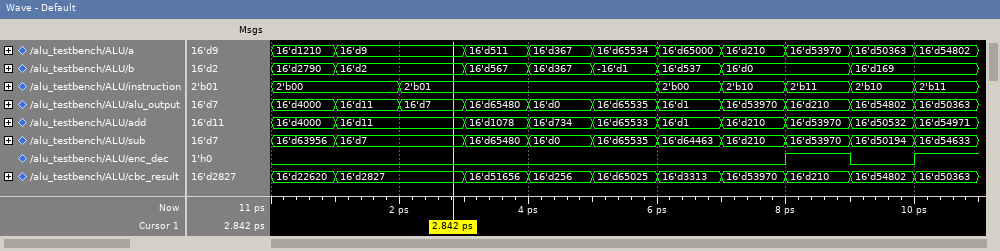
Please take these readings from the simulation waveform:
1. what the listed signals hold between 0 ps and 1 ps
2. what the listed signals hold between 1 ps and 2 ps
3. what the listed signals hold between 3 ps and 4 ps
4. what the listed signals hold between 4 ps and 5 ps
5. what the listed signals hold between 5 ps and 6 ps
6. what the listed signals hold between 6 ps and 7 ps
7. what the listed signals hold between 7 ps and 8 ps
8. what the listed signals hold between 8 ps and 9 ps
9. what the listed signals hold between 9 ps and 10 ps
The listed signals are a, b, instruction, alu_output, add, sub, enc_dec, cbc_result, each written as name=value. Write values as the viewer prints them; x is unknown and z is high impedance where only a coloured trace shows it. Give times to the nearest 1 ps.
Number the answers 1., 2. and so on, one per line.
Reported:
1. a=16'd1210, b=16'd2790, instruction=2'b00, alu_output=16'd4000, add=16'd4000, sub=16'd63956, enc_dec=0, cbc_result=16'd22620
2. a=16'd9, b=16'd2, instruction=2'b00, alu_output=16'd11, add=16'd11, sub=16'd7, enc_dec=0, cbc_result=16'd2827
3. a=16'd511, b=16'd567, instruction=2'b01, alu_output=16'd65480, add=16'd1078, sub=16'd65480, enc_dec=0, cbc_result=16'd51656
4. a=16'd367, b=16'd367, instruction=2'b01, alu_output=16'd0, add=16'd734, sub=16'd0, enc_dec=0, cbc_result=16'd256
5. a=16'd65534, b=-16'd1, instruction=2'b01, alu_output=16'd65535, add=16'd65533, sub=16'd65535, enc_dec=0, cbc_result=16'd65025
6. a=16'd65000, b=16'd537, instruction=2'b00, alu_output=16'd1, add=16'd1, sub=16'd64463, enc_dec=0, cbc_result=16'd3313
7. a=16'd210, b=16'd0, instruction=2'b10, alu_output=16'd53970, add=16'd210, sub=16'd210, enc_dec=0, cbc_result=16'd53970
8. a=16'd53970, b=16'd0, instruction=2'b11, alu_output=16'd210, add=16'd53970, sub=16'd53970, enc_dec=1, cbc_result=16'd210
9. a=16'd50363, b=16'd169, instruction=2'b10, alu_output=16'd54802, add=16'd50532, sub=16'd50194, enc_dec=0, cbc_result=16'd54802
